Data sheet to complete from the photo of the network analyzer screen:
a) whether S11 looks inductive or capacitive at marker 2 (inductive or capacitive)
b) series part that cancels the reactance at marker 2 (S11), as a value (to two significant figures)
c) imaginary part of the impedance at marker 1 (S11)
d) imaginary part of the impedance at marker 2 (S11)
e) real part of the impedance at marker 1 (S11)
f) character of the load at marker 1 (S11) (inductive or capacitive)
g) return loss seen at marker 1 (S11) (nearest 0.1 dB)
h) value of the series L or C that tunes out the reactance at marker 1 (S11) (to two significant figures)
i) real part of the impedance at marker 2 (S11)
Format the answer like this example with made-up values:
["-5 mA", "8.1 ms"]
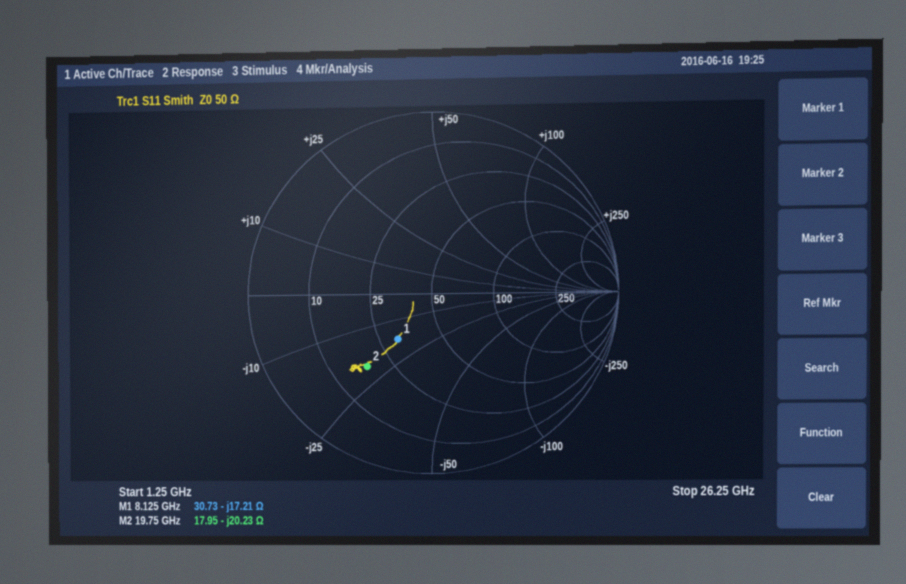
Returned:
["capacitive", "160 pH", "-17.21 Ω", "-20.23 Ω", "30.73 Ω", "capacitive", "10.1 dB", "340 pH", "17.95 Ω"]
